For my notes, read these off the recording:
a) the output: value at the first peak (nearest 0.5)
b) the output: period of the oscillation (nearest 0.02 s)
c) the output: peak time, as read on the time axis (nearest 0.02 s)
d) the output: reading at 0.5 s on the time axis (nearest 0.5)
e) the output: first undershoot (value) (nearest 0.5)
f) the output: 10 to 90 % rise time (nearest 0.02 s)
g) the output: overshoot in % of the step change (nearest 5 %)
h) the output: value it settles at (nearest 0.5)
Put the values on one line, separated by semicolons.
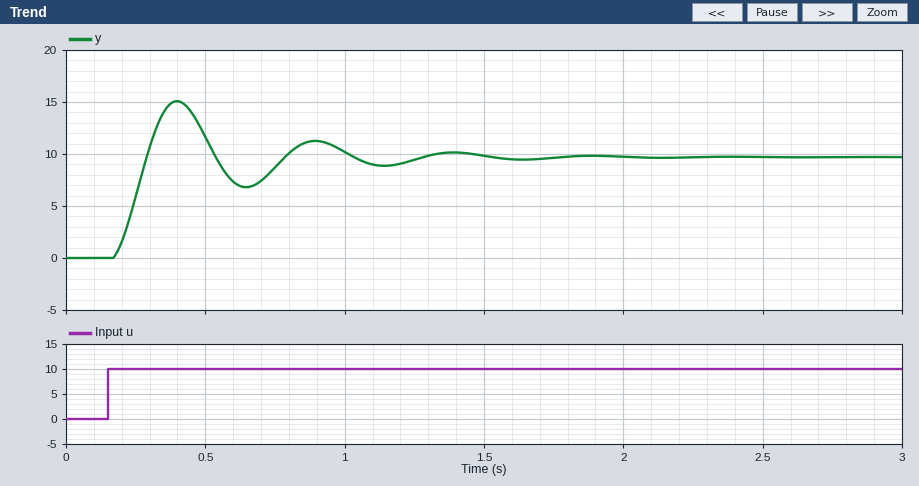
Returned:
15.0; 0.50 s; 0.40 s; 11.5; 7.0; 0.08 s; 55 %; 9.5
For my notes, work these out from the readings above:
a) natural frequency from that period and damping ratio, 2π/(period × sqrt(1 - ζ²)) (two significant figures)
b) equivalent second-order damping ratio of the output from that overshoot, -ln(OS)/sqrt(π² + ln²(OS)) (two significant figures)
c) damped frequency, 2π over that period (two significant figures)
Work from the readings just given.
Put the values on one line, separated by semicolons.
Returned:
13 rad/s; 0.19; 13 rad/s
